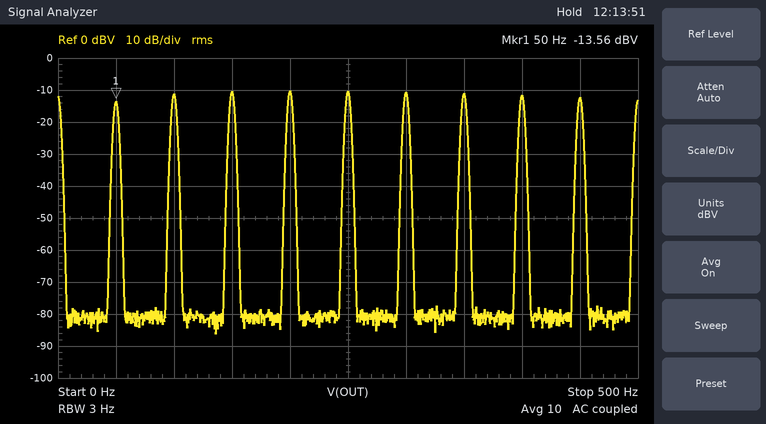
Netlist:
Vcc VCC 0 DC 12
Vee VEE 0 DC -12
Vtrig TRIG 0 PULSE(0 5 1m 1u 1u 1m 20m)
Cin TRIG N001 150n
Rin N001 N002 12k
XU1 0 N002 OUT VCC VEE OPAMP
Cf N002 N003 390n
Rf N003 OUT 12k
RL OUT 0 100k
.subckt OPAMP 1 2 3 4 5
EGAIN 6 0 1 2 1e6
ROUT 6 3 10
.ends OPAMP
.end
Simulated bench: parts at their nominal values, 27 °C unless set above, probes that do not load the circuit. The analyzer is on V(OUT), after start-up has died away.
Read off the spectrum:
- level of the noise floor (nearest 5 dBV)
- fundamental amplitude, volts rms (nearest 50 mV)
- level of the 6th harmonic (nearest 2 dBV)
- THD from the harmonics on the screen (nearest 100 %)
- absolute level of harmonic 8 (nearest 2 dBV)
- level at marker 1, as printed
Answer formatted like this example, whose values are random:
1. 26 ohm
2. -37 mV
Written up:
1. -80 dBV
2. 200 mV
3. -10 dBV
4. 400 %
5. -12 dBV
6. -13.56 dBV
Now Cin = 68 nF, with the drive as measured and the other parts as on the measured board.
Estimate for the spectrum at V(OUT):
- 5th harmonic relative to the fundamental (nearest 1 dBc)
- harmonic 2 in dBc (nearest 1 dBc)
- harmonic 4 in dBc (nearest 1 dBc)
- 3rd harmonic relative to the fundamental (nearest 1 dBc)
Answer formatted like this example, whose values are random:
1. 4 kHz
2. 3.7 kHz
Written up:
1. 8 dBc
2. 4 dBc
3. 7 dBc
4. 6 dBc
